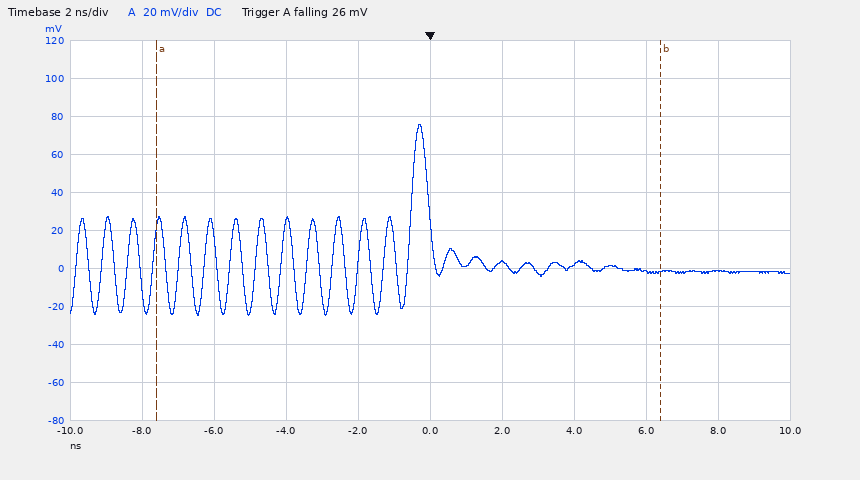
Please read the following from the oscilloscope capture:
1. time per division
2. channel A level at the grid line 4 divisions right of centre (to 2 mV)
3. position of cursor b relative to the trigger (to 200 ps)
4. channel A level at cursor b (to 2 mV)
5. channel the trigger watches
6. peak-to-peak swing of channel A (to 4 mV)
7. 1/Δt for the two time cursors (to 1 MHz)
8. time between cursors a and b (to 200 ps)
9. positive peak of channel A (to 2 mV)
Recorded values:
2 ns
-2 mV
+6.4 ns
-2 mV
channel A
100 mV
71 MHz
14.0 ns
76 mV
